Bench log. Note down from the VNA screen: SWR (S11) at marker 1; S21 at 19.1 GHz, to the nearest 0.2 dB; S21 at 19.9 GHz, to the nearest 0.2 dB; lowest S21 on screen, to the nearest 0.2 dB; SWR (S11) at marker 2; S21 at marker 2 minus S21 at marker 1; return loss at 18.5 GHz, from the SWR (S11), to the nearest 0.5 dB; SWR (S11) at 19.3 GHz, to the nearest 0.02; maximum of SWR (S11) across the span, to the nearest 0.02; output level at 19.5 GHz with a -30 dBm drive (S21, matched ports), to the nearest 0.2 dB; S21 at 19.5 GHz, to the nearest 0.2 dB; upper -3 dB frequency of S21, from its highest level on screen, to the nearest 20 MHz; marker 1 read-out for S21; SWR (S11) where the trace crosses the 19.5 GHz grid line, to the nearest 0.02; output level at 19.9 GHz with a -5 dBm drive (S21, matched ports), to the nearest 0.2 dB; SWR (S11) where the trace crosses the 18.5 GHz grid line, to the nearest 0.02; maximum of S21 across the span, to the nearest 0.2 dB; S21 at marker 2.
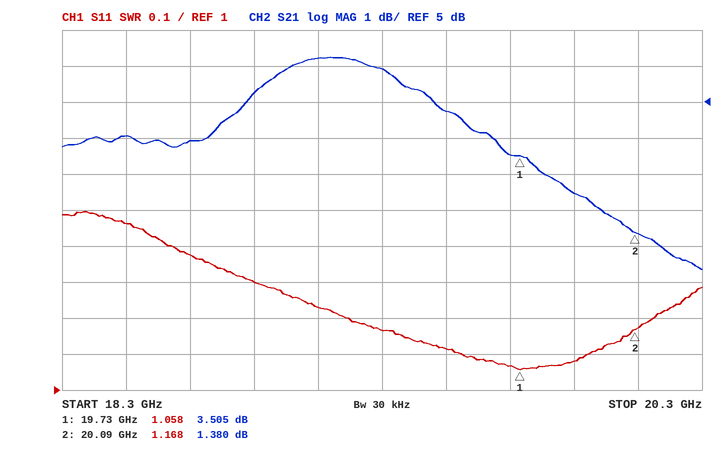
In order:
1.058
6.2 dB
2.4 dB
0.4 dB
1.168
-2.125 dB
14.5 dB
1.16
1.50
-25.2 dBm
4.8 dB
19.78 GHz
3.505 dB
1.12
-2.6 dBm
1.46
6.2 dB
1.380 dB
